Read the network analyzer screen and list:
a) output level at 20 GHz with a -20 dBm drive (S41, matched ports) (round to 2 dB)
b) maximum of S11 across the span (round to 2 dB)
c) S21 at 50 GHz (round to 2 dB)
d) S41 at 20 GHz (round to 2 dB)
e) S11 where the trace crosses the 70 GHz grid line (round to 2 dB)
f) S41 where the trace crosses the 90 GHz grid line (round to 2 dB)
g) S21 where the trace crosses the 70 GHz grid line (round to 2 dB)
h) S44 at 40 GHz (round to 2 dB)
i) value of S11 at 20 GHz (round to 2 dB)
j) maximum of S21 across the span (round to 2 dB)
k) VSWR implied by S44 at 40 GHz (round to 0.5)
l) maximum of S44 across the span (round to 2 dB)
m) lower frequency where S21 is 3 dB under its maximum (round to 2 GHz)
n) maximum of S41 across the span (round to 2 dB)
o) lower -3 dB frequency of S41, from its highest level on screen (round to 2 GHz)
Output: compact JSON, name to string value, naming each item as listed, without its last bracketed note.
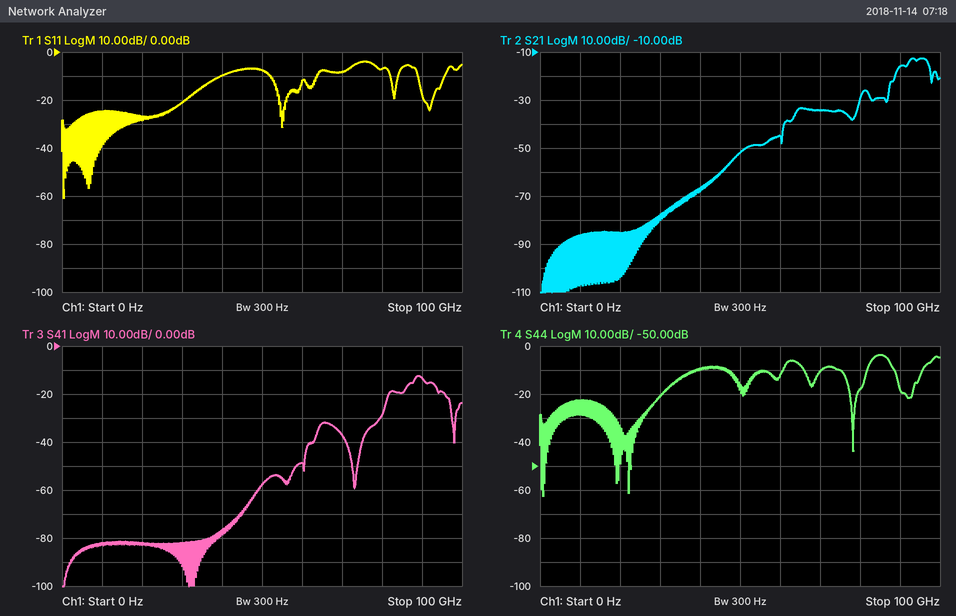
{"output level at 20 GHz with a -20 dBm drive (S41, matched ports)": "-102 dBm", "maximum of S11 across the span": "-4 dB", "S21 at 50 GHz": "-52 dB", "S41 at 20 GHz": "-82 dB", "S11 where the trace crosses the 70 GHz grid line": "-8 dB", "S41 where the trace crosses the 90 GHz grid line": "-14 dB", "S21 where the trace crosses the 70 GHz grid line": "-34 dB", "S44 at 40 GHz": "-10 dB", "value of S11 at 20 GHz": "-28 dB", "maximum of S21 across the span": "-12 dB", "VSWR implied by S44 at 40 GHz": "2.0", "maximum of S44 across the span": "-4 dB", "lower frequency where S21 is 3 dB under its maximum": "92 GHz", "maximum of S41 across the span": "-12 dB", "lower -3 dB frequency of S41, from its highest level on screen": "88 GHz"}
